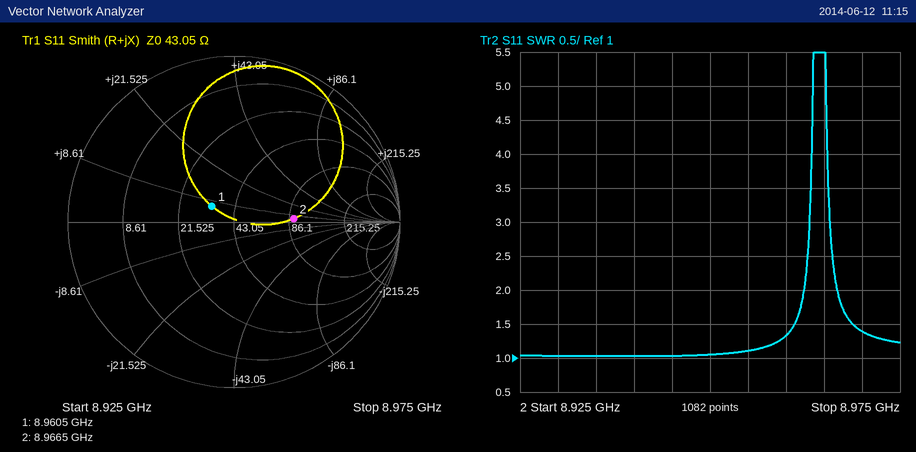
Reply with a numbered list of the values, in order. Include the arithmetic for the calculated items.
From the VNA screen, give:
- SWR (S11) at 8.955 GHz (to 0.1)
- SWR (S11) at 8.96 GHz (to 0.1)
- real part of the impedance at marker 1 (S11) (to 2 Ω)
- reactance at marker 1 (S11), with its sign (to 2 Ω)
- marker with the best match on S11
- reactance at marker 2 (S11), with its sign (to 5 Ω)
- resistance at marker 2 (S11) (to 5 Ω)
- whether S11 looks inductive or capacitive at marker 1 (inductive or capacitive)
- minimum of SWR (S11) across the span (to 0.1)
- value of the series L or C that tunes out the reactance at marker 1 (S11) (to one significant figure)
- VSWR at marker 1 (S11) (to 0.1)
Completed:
1. 1.1
2. 1.3
3. 32 Ω
4. +6 Ω
5. marker 1
6. +5 Ω
7. 90 Ω
8. inductive
9. 1.0
10. C = 1/(2π × 8.9605 GHz × 6 Ω) ≈ 3 pF
11. 1.4
